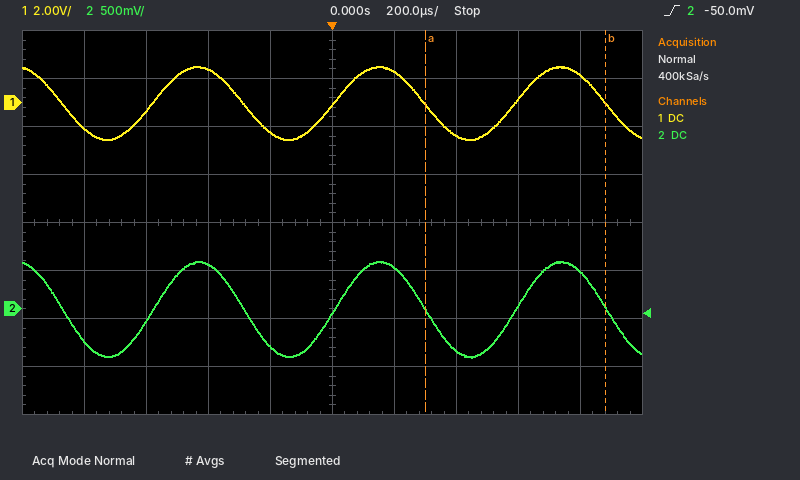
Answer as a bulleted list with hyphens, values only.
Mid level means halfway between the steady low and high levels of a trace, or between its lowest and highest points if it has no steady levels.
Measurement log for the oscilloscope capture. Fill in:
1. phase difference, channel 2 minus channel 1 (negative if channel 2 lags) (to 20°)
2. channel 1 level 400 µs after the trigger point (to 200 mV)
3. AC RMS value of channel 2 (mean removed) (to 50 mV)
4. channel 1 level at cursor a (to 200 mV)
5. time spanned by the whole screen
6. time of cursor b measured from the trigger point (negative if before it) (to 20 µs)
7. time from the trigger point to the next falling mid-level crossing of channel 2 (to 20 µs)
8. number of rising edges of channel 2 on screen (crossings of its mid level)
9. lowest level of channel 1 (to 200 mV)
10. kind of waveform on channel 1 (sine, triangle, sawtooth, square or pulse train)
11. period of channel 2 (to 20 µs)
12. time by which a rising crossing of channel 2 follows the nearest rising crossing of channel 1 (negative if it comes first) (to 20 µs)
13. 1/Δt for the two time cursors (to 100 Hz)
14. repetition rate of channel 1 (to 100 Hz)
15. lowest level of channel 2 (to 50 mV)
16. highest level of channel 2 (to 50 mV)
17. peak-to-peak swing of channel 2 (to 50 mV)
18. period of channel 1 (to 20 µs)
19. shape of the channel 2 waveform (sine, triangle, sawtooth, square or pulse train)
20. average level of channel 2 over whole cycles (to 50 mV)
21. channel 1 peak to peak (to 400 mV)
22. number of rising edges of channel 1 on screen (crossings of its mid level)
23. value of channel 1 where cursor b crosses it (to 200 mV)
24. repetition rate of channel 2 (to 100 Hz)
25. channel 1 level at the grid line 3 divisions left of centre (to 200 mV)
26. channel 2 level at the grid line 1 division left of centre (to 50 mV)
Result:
- 0°
- -1.4 V
- 350 mV
- 0.0 V
- 2 ms
- +880 µs
- 300 µs
- 3
- -1.6 V
- sine
- 580 µs
- 0 µs
- 1.7 kHz
- 1.7 kHz
- -500 mV
- 500 mV
- 1.00 V
- 580 µs
- sine
- 0 mV
- 3.2 V
- 3
- 0.0 V
- 1.7 kHz
- -400 mV
- -400 mV
